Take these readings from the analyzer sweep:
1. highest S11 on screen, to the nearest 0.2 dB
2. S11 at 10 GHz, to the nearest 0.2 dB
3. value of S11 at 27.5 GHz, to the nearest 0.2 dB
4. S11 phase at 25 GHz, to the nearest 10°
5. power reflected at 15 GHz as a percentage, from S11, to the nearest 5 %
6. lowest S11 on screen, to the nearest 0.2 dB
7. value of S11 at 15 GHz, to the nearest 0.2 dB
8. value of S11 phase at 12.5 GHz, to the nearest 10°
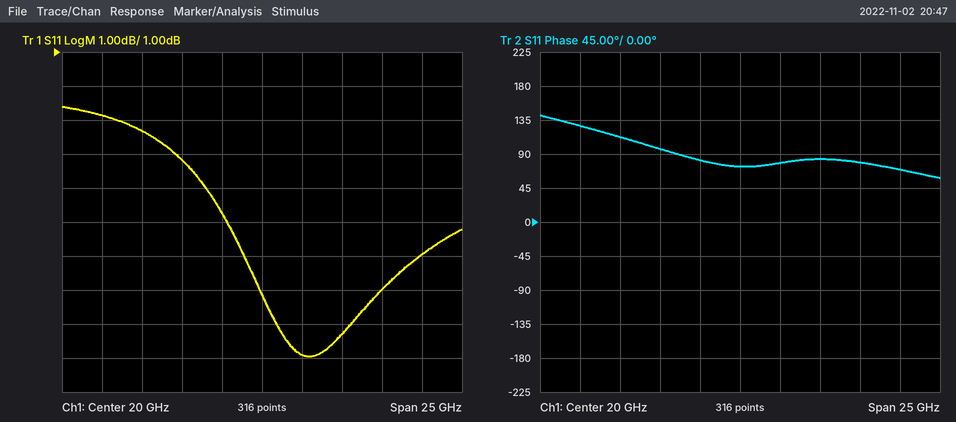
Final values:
-0.6 dB
-0.8 dB
-6.0 dB
80°
60 %
-8.0 dB
-2.2 dB
110°
